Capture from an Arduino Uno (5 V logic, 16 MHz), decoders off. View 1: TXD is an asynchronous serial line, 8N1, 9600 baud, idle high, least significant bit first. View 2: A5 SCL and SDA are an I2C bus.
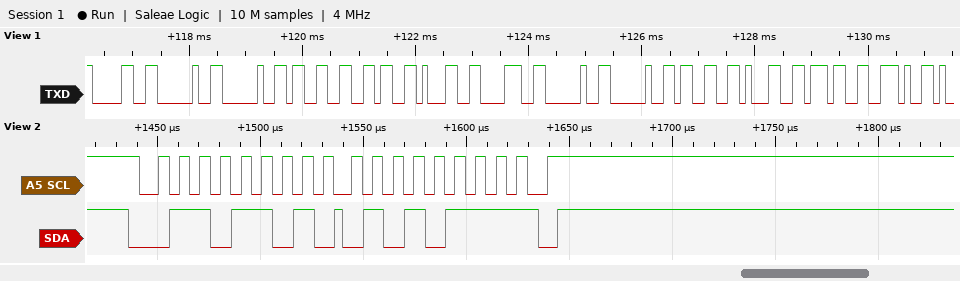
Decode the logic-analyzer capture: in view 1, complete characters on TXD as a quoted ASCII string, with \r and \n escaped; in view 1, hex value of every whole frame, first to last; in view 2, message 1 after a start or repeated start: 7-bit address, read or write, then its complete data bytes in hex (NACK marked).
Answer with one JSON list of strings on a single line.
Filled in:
["\"0  3618  317.\"", "30 20 20 33 36 31 38 20 20 33 31 37 2E", "0x36 read: 57 NACK"]
